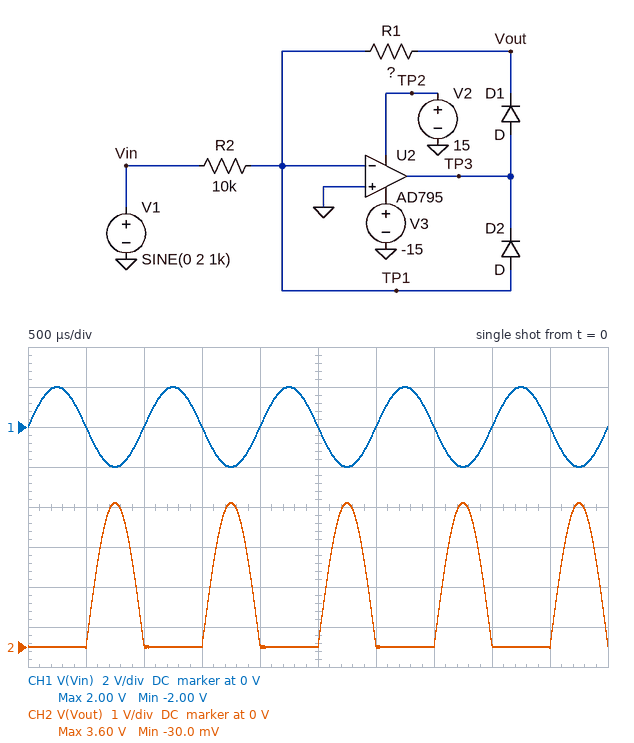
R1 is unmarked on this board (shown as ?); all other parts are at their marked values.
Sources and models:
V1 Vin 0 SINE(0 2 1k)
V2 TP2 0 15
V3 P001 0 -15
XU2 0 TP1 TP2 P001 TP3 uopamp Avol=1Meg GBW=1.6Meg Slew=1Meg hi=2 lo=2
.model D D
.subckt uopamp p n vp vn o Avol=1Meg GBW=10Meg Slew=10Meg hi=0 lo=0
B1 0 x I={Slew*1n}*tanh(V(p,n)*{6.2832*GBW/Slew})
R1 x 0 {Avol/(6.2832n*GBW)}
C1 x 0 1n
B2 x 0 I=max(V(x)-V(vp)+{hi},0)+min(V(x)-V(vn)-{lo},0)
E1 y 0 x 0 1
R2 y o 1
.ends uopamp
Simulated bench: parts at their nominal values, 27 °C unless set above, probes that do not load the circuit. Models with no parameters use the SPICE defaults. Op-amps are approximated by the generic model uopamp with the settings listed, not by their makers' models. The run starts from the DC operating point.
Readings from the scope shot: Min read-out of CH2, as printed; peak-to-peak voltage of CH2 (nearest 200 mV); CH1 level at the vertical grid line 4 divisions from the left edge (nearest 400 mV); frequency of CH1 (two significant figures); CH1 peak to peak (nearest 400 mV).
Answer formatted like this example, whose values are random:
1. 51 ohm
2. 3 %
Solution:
1. -30.0 mV
2. 3.6 V
3. 0 V
4. 1.0 kHz
5. 4.0 V
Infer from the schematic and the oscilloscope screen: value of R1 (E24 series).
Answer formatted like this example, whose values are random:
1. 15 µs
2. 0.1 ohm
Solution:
1. 18 kΩ
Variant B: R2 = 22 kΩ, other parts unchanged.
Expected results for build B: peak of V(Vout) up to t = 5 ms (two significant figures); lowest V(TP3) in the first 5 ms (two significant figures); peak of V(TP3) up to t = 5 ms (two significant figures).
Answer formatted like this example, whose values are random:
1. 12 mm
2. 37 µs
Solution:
1. 1.6 V
2. -590 mV
3. 2.2 V
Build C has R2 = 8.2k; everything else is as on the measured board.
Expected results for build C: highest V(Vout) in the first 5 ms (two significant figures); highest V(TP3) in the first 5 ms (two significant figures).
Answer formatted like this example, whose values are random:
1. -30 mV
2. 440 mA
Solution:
1. 4.4 V
2. 5.0 V
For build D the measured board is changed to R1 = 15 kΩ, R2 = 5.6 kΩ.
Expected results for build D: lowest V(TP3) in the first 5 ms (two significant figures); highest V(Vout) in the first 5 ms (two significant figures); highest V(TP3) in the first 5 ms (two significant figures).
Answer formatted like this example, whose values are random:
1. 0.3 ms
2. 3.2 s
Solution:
1. -630 mV
2. 5.4 V
3. 6.0 V
